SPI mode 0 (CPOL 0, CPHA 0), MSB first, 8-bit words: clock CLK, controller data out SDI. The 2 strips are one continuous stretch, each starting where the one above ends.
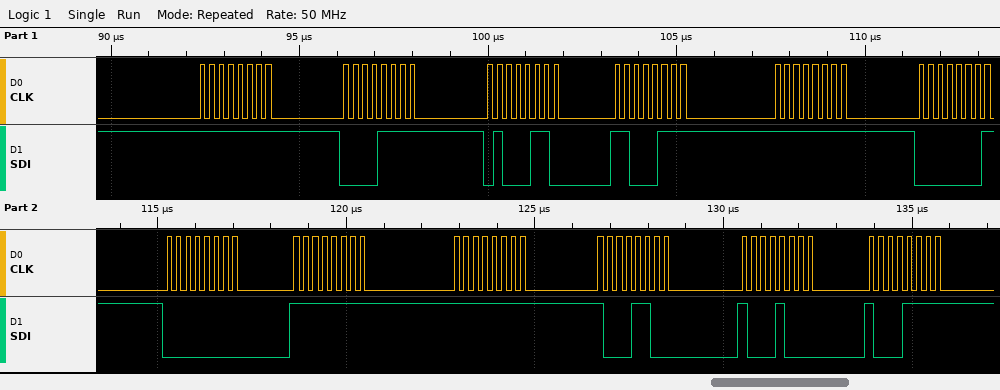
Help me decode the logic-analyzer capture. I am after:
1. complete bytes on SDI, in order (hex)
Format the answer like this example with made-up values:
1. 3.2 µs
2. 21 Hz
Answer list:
1. FF 0F 46 C7 FF 01 00 FF FF 8C 88 8F
